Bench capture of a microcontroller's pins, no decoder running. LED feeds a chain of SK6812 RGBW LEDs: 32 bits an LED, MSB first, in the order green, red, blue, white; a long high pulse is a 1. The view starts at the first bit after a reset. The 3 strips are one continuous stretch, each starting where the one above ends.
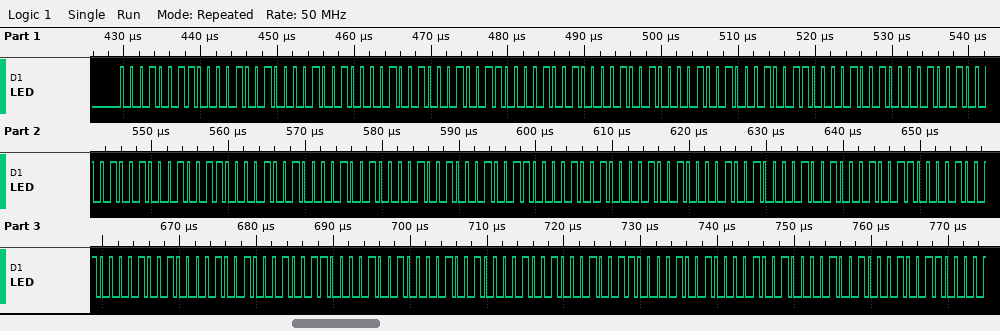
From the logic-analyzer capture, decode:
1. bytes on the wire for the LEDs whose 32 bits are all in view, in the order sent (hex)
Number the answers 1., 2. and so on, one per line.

1. 13 09 09 09 13 09 09 09 13 09 09 09 13 09 09 09 13 09 09 09 09 13 09 09 09 13 09 09 09 13 09 09
